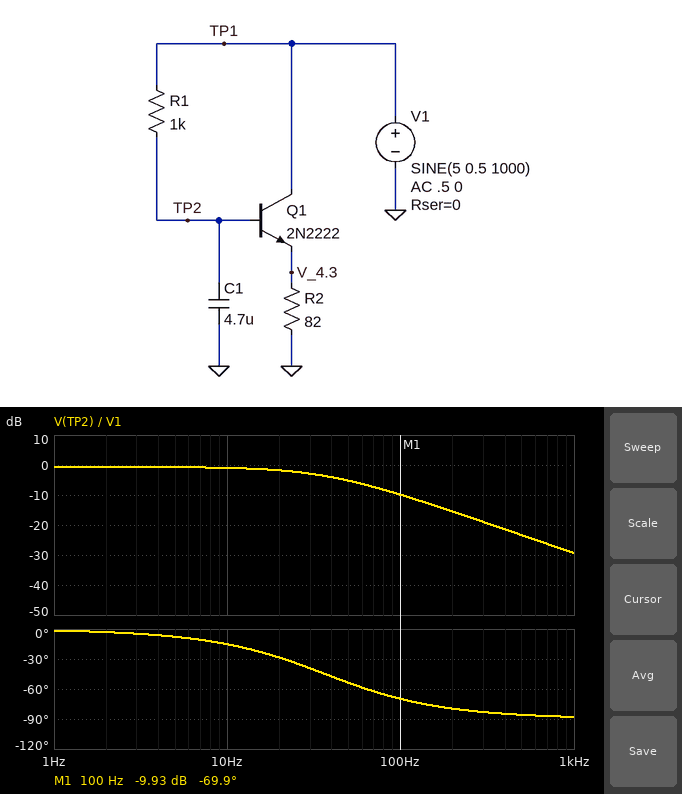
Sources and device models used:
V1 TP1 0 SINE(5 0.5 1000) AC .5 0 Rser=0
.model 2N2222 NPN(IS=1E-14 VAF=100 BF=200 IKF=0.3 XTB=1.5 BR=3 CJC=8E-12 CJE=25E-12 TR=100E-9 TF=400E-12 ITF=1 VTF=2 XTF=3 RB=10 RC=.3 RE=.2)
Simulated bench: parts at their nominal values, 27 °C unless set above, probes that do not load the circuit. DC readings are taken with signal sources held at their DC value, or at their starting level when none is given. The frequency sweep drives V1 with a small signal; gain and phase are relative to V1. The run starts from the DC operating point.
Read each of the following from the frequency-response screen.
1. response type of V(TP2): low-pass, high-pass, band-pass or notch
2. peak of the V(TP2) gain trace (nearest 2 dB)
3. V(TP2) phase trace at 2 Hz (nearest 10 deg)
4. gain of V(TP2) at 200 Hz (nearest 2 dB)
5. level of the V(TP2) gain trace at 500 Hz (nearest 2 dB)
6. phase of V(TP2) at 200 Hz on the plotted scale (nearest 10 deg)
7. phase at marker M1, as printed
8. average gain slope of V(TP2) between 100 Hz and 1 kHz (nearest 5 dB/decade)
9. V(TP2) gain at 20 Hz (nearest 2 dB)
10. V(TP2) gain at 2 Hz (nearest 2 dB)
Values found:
low-pass
0 dB
0 deg
-16 dB
-24 dB
-80 deg
-69.9 deg
-20 dB/decade
-2 dB
0 dB
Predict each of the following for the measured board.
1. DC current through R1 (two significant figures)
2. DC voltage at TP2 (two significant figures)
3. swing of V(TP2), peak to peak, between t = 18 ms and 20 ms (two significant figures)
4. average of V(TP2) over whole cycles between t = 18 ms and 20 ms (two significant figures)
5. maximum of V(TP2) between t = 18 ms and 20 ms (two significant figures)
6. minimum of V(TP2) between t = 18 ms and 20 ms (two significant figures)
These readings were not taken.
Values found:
280 µA
4.7 V
34 mV
4.7 V
4.7 V
4.7 V
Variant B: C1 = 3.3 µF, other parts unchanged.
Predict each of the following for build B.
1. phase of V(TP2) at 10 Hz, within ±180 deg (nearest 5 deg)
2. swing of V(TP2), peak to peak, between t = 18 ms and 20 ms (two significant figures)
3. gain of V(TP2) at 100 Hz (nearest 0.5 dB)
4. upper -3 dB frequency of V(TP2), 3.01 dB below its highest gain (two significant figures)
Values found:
-10 deg
48 mV
-7.5 dB
52 Hz
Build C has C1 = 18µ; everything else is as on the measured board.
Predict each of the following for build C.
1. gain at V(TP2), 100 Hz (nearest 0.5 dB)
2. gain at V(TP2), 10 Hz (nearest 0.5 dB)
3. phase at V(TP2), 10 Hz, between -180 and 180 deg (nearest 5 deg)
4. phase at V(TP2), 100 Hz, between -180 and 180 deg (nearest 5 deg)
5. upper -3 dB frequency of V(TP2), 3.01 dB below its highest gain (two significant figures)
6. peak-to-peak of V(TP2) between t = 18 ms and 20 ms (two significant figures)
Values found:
-21.0 dB
-4.0 dB
-45 deg
-85 deg
9.6 Hz
9.0 mV
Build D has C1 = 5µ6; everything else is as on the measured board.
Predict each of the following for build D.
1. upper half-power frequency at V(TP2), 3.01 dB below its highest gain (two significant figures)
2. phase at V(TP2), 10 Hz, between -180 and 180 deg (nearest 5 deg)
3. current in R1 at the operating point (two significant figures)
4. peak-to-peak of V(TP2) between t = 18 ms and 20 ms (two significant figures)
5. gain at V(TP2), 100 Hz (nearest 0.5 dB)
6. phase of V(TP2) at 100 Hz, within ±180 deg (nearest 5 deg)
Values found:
31 Hz
-20 deg
280 µA
29 mV
-11.5 dB
-75 deg
